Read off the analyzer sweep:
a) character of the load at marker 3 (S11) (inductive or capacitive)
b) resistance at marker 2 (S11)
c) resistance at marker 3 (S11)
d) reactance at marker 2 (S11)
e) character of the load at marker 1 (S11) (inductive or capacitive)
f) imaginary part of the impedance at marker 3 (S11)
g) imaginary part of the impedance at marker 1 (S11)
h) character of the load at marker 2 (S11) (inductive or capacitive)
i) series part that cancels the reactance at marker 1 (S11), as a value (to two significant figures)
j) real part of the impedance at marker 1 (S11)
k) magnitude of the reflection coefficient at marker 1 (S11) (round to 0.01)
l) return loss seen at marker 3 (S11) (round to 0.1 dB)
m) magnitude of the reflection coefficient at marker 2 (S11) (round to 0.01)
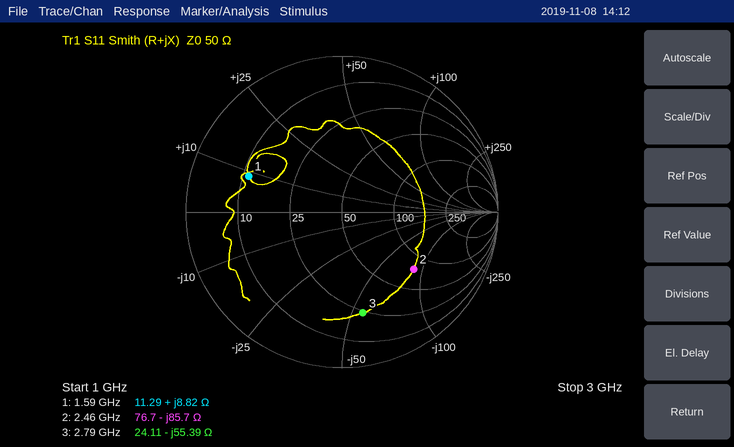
capacitive
76.7 Ω
24.11 Ω
-85.7 Ω
inductive
-55.39 Ω
+8.82 Ω
capacitive
11 pF
11.29 Ω
0.64
3.6 dB
0.59
